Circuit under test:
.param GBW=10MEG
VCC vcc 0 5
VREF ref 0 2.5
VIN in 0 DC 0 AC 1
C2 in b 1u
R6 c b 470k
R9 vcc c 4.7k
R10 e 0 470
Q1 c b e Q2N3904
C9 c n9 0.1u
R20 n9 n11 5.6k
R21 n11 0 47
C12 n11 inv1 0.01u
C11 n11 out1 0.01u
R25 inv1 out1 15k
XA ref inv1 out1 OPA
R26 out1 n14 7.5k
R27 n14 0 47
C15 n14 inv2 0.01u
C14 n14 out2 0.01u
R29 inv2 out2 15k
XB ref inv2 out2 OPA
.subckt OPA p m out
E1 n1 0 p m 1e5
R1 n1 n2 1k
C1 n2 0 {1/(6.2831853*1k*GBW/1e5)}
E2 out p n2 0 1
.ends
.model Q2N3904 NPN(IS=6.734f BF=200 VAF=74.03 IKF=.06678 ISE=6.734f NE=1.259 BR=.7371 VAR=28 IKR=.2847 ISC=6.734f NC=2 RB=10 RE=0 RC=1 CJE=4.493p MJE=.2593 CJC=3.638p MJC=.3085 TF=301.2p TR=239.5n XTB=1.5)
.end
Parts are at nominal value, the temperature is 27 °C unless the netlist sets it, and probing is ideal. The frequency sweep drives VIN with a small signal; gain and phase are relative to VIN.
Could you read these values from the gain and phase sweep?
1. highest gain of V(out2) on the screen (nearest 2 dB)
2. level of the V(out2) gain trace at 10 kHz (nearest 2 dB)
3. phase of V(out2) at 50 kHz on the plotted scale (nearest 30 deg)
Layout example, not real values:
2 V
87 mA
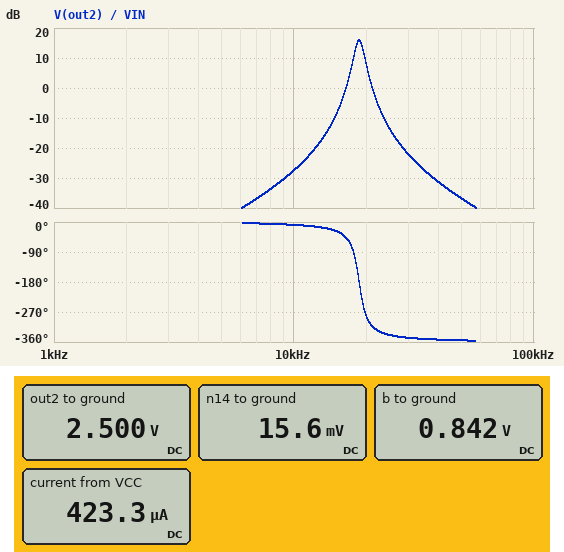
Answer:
16 dB
-28 dB
-360 deg
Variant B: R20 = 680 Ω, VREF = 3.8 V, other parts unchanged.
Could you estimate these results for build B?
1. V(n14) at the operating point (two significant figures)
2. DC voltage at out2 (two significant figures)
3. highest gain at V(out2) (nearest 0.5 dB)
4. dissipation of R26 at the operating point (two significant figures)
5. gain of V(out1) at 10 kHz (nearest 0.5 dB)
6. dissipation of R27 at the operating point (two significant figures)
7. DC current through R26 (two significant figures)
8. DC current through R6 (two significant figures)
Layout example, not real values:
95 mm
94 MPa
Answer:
24 mV
3.8 V
21.5 dB
1.9 mW
0 dB
12 µW
500 µA
4.6 µA
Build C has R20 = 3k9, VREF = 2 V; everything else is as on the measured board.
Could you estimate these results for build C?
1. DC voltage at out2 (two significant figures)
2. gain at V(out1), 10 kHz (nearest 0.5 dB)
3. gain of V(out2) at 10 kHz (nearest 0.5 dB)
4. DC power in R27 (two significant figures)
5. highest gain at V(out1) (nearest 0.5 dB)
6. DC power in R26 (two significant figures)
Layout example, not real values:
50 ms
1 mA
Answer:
2.0 V
-4.0 dB
-26.0 dB
3.3 µW
17.5 dB
530 µW
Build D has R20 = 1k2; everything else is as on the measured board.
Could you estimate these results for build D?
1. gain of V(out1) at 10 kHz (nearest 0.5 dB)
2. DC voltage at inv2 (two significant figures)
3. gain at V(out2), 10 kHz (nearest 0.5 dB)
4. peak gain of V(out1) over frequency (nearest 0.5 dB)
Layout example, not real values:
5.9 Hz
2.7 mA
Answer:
-1.0 dB
2.5 V
-22.5 dB
21.0 dB
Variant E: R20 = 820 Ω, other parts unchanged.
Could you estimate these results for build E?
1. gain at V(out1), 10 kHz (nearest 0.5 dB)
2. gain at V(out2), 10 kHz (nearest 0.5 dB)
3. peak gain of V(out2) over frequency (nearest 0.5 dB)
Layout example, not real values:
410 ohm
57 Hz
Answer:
-0.5 dB
-22.0 dB
21.5 dB
